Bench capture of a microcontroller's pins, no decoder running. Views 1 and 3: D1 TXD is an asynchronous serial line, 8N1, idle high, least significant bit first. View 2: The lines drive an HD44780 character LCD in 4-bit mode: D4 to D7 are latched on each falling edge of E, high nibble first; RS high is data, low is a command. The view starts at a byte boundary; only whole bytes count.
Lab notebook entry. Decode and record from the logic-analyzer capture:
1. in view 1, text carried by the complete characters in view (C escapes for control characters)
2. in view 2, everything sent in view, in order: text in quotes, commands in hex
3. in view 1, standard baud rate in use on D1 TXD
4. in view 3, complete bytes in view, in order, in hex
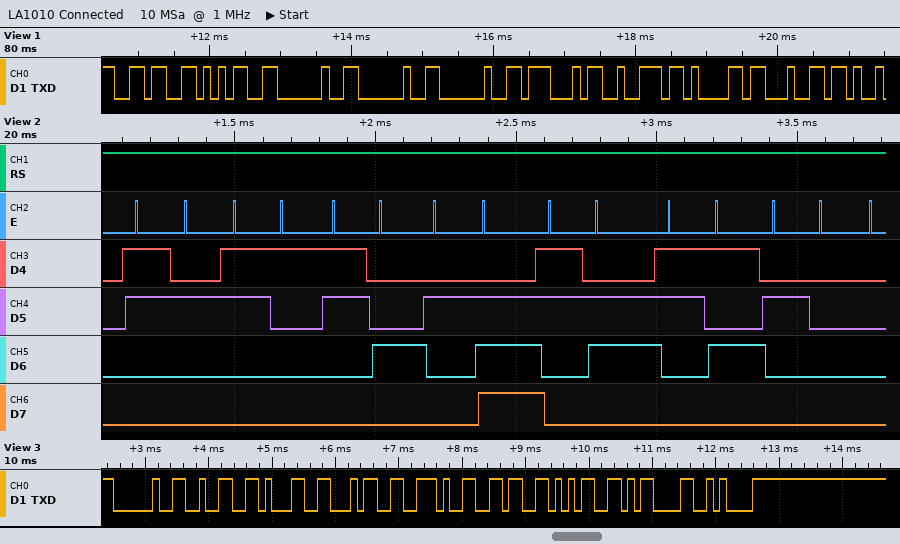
"65   Grad"
"214.65 "
9600 baud
20 32 31 34 2E 36 35 0D 0A
